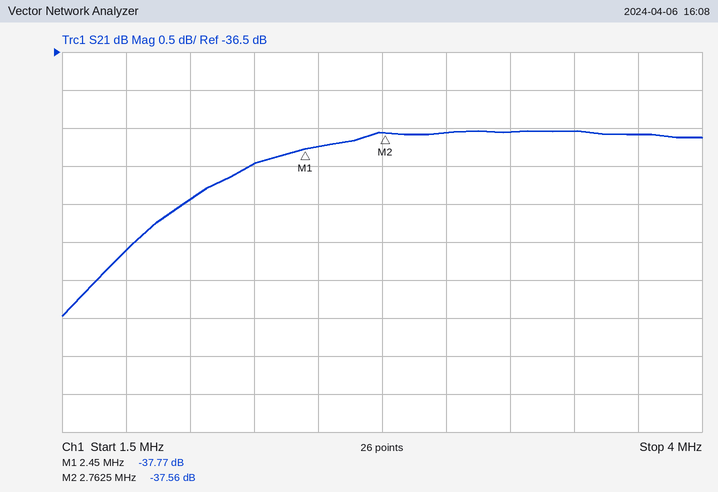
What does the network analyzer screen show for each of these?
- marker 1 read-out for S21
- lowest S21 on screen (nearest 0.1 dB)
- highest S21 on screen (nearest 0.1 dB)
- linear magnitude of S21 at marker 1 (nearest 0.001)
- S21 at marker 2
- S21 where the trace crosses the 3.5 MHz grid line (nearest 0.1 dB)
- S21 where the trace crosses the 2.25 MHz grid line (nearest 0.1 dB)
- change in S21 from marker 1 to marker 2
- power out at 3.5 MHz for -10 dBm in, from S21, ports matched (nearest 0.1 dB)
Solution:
-37.77 dB
-40.0 dB
-37.5 dB
0.013
-37.56 dB
-37.5 dB
-38.0 dB
0.21 dB
-47.5 dBm
